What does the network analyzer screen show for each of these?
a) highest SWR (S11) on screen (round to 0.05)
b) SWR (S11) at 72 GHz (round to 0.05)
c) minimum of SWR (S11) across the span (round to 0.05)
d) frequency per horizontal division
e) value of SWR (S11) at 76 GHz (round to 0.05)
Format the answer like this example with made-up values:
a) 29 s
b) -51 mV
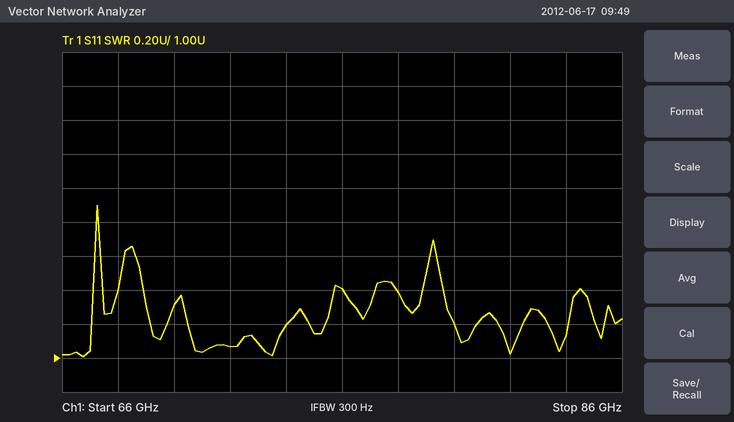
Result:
a) 1.90
b) 1.05
c) 1.00
d) 2 GHz
e) 1.40
